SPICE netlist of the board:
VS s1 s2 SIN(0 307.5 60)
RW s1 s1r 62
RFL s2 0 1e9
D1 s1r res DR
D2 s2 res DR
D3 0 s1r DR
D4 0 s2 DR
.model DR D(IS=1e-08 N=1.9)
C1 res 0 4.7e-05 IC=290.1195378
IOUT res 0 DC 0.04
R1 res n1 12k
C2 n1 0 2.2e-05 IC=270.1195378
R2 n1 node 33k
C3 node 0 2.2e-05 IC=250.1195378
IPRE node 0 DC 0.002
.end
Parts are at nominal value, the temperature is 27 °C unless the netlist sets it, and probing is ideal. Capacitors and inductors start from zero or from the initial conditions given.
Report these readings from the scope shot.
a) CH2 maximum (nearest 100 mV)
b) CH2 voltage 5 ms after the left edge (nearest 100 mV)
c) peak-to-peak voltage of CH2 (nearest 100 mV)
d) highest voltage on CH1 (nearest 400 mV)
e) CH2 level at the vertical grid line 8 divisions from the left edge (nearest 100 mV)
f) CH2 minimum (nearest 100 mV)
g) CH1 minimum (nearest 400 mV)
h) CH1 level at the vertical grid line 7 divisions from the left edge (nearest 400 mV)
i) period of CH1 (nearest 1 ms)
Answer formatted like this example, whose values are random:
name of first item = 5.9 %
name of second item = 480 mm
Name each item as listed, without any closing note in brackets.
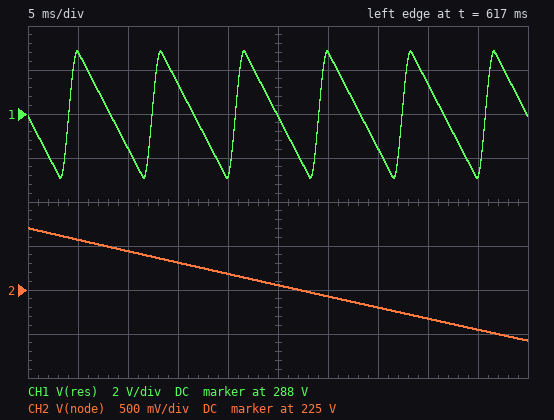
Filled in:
CH2 maximum = 225.7 V
CH2 voltage 5 ms after the left edge = 225.6 V
peak-to-peak voltage of CH2 = 1.3 V
highest voltage on CH1 = 290.8 V
CH2 level at the vertical grid line 8 divisions from the left edge = 224.7 V
CH2 minimum = 224.4 V
CH1 minimum = 285.2 V
CH1 level at the vertical grid line 7 divisions from the left edge = 286.4 V
period of CH1 = 8 ms
